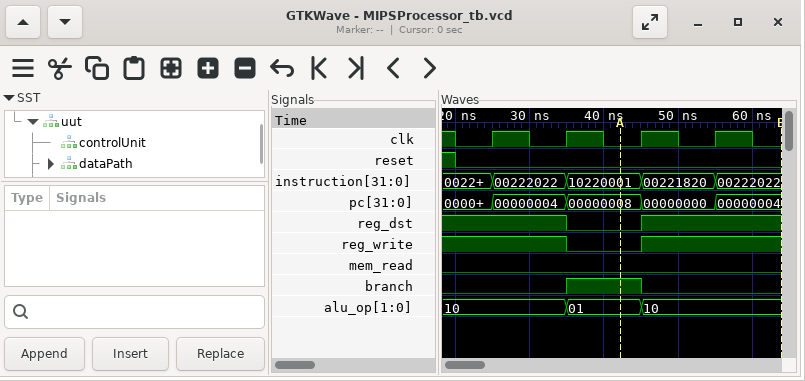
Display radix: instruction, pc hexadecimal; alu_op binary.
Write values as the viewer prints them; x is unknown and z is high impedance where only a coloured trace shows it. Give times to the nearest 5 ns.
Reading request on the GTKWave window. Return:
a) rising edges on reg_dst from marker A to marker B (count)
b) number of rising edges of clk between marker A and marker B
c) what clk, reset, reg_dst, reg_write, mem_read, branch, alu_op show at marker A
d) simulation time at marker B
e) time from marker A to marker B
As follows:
1
2
clk=0, reset=0, reg_dst=0, reg_write=0, mem_read=0, branch=1, alu_op=01
65 ns
20 ns
